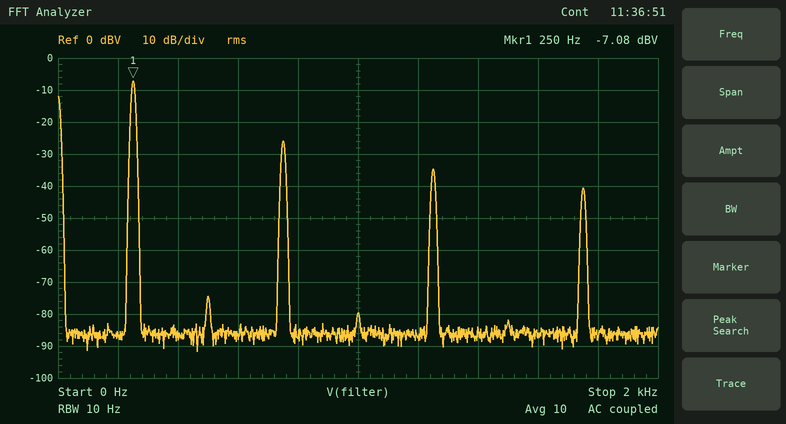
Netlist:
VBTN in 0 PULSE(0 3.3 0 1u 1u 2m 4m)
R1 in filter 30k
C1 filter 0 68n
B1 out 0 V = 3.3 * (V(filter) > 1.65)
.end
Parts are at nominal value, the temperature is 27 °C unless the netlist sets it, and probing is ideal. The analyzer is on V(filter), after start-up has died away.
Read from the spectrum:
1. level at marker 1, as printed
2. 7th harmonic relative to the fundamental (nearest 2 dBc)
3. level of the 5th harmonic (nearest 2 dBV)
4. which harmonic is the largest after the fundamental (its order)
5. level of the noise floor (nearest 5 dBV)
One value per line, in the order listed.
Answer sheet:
-7.08 dBV
-34 dBc
-34 dBV
3
-85 dBV
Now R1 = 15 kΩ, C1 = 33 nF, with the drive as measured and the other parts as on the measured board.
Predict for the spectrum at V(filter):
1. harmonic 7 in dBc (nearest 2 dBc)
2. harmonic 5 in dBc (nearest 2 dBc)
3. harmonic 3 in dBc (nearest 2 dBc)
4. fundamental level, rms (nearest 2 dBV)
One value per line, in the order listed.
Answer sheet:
-30 dBc
-24 dBc
-16 dBc
2 dBV
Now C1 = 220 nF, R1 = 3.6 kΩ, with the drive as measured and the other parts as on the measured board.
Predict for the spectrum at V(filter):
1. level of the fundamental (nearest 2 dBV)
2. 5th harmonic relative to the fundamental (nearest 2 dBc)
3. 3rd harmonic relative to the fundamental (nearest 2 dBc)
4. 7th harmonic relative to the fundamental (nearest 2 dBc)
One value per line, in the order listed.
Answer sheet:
0 dBV
-26 dBc
-18 dBc
-32 dBc
